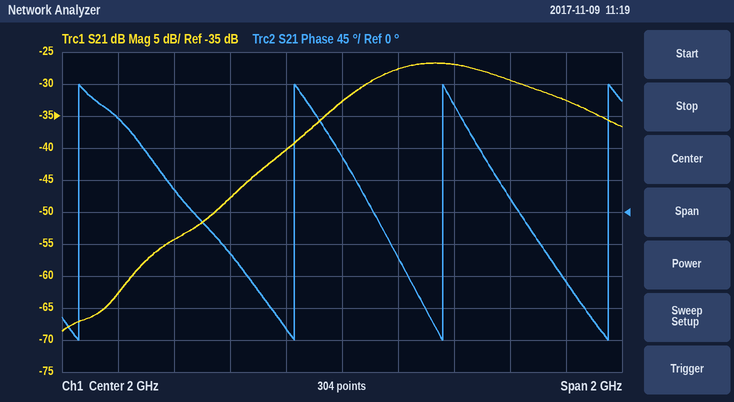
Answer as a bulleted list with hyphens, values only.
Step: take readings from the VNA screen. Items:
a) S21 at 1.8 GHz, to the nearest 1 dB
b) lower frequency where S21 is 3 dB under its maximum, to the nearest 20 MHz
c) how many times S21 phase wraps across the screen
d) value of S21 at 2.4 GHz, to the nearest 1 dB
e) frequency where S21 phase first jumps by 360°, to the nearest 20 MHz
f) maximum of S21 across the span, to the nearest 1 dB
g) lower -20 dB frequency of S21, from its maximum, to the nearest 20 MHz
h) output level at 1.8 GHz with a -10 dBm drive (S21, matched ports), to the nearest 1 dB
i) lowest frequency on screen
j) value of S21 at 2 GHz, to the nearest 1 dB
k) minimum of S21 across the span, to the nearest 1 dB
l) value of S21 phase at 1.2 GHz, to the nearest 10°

- -40 dB
- 2.10 GHz
- 4
- -27 dB
- 1.06 GHz
- -27 dB
- 1.62 GHz
- -50 dBm
- 1 GHz
- -33 dB
- -69 dB
- 130°
